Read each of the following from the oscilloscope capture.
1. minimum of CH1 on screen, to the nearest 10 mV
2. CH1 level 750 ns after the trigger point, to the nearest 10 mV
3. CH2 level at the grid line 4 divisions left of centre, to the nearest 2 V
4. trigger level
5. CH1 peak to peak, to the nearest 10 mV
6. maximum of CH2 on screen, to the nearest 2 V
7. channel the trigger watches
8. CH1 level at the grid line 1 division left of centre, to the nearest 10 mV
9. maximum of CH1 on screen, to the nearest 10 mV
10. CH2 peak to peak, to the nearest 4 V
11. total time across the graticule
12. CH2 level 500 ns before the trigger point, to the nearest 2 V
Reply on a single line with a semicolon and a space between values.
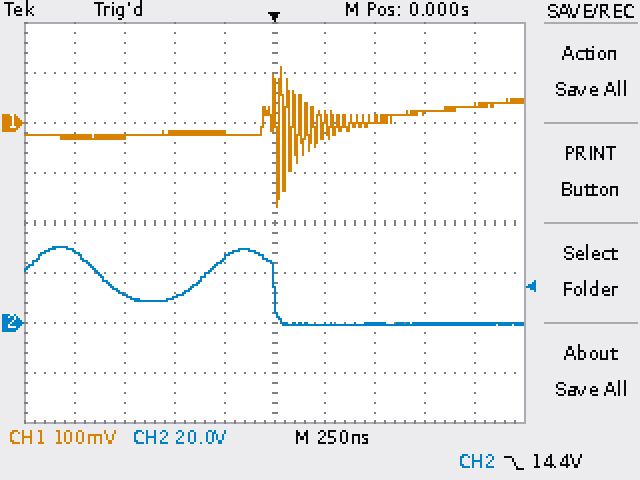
-170 mV; 20 mV; 28 V; 14.4 V; 280 mV; 30 V; CH2; -20 mV; 110 mV; 32 V; 2.5 µs; 10 V
